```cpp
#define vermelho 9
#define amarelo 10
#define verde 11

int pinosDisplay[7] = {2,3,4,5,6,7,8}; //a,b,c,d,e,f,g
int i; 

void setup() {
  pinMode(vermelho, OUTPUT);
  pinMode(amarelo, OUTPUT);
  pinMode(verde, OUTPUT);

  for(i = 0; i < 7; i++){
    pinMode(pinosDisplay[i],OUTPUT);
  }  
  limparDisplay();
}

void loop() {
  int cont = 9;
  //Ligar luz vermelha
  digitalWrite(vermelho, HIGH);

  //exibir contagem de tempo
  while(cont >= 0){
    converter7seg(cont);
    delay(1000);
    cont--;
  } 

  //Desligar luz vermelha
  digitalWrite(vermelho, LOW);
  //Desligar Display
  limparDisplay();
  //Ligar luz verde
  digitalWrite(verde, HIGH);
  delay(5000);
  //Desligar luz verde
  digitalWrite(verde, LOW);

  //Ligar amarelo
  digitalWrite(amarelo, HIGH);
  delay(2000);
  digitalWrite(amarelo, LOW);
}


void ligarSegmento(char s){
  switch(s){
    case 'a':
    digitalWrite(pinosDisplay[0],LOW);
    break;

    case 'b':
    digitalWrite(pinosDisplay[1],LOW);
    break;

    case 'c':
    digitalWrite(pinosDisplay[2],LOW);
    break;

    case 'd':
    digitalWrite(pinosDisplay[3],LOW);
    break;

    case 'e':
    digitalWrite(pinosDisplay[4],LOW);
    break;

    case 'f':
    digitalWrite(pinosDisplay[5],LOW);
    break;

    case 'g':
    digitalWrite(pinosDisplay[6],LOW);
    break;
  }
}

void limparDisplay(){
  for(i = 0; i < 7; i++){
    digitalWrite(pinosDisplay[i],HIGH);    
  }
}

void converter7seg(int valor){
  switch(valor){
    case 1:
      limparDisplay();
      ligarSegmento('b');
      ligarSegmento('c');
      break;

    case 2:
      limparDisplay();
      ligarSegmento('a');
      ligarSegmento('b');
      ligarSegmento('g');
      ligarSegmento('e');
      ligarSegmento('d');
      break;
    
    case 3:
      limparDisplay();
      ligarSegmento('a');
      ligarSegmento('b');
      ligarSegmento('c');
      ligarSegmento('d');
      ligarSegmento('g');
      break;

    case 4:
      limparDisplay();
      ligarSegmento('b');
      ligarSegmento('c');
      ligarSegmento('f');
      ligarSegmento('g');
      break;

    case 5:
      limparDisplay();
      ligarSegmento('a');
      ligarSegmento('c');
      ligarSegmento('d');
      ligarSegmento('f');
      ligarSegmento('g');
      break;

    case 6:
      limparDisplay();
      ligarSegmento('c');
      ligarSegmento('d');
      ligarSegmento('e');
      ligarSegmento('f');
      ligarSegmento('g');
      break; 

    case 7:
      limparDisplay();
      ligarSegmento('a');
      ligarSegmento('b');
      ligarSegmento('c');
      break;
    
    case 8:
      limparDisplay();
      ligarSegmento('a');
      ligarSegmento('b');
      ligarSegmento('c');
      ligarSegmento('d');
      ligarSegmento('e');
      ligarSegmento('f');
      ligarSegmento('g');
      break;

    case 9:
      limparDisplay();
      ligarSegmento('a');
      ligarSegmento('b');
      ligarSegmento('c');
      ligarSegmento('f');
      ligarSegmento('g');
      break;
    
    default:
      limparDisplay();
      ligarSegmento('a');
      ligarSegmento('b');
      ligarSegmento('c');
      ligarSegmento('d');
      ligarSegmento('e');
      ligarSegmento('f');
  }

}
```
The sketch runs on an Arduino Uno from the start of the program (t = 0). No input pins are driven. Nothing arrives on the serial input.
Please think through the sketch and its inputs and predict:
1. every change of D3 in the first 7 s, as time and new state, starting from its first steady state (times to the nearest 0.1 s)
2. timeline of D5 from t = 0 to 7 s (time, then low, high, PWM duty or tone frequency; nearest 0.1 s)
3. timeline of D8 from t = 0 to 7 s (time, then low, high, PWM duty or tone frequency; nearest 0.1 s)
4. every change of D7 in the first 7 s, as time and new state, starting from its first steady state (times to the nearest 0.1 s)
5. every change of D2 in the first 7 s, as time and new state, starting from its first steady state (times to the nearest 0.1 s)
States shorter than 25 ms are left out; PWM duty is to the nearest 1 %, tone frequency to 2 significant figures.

0 s low; 3 s high; 5 s low
0 s high; 1 s low; 2 s high; 3 s low; 5 s high; 6 s low
0 s low; 2 s high; 3 s low
0 s low; 2 s high; 3 s low; 6 s high
0 s low; 3 s high; 4 s low; 5 s high; 6 s low
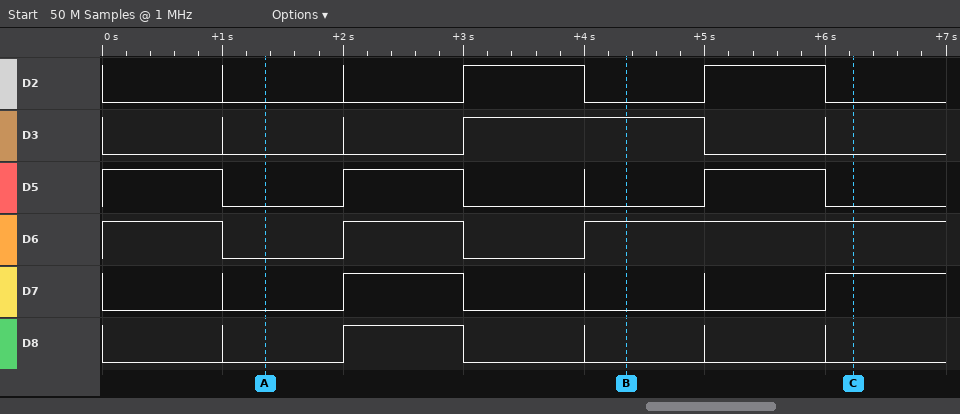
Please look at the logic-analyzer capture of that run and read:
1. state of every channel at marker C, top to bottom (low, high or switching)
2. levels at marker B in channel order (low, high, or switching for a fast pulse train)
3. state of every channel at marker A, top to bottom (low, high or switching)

D2 low, D3 low, D5 low, D6 high, D7 high, D8 low
D2 low, D3 high, D5 low, D6 high, D7 low, D8 low
D2 low, D3 low, D5 low, D6 low, D7 low, D8 low
